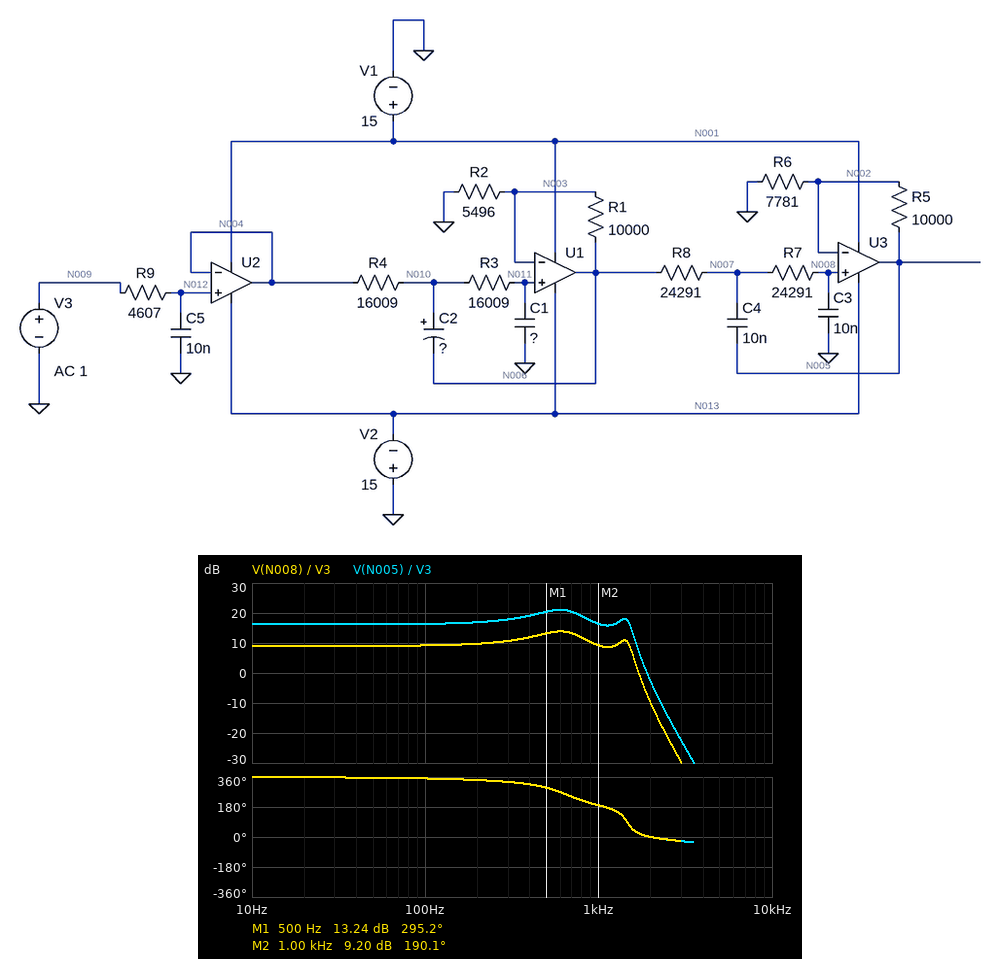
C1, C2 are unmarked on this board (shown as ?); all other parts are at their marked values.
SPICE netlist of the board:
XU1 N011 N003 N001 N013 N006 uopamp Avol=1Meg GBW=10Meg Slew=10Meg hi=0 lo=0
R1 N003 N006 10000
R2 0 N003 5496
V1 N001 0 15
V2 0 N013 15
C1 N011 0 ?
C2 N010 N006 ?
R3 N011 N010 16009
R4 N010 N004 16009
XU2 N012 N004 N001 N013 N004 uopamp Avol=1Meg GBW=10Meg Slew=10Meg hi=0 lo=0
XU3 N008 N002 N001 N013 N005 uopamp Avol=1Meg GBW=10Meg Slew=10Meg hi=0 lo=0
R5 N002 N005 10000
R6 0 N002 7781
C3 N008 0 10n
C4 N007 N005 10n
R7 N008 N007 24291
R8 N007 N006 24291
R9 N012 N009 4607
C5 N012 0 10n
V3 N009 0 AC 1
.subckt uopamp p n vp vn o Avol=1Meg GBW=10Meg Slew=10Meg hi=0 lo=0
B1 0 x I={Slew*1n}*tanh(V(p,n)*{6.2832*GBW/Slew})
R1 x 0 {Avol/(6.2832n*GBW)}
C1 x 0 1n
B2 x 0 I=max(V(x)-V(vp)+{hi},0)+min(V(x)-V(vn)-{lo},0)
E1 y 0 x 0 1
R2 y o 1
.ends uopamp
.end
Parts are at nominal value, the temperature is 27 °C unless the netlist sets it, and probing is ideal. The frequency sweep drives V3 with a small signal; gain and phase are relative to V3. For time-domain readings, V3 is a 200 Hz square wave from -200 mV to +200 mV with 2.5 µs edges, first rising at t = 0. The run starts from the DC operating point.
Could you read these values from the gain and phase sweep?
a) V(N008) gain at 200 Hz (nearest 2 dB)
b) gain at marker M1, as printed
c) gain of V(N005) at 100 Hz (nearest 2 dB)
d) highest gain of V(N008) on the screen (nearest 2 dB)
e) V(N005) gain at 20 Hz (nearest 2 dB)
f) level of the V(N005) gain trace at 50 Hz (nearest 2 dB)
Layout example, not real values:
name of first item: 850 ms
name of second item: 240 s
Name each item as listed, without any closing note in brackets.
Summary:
V(N008) gain at 200 Hz: 10 dB
gain at marker M1, as printed: 13.24 dB
gain of V(N005) at 100 Hz: 16 dB
highest gain of V(N008) on the screen: 14 dB
V(N005) gain at 20 Hz: 16 dB
level of the V(N005) gain trace at 50 Hz: 16 dB
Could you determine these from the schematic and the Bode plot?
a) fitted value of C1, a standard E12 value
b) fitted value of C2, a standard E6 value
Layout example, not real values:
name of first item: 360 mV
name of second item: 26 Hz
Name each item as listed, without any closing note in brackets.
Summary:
fitted value of C1, a standard E12 value: 6.8 nF
fitted value of C2, a standard E6 value: 6.8 nF
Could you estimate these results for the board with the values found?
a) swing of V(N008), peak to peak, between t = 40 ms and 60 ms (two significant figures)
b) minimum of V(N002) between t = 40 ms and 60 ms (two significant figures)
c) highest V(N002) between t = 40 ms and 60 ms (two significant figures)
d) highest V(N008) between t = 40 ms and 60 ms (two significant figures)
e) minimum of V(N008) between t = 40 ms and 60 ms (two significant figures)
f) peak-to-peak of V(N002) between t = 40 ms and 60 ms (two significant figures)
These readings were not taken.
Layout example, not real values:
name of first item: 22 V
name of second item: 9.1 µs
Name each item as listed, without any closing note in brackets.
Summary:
swing of V(N008), peak to peak, between t = 40 ms and 60 ms: 2.2 V
minimum of V(N002) between t = 40 ms and 60 ms: -1.1 V
highest V(N002) between t = 40 ms and 60 ms: 1.1 V
highest V(N008) between t = 40 ms and 60 ms: 1.1 V
minimum of V(N008) between t = 40 ms and 60 ms: -1.1 V
peak-to-peak of V(N002) between t = 40 ms and 60 ms: 2.2 V
